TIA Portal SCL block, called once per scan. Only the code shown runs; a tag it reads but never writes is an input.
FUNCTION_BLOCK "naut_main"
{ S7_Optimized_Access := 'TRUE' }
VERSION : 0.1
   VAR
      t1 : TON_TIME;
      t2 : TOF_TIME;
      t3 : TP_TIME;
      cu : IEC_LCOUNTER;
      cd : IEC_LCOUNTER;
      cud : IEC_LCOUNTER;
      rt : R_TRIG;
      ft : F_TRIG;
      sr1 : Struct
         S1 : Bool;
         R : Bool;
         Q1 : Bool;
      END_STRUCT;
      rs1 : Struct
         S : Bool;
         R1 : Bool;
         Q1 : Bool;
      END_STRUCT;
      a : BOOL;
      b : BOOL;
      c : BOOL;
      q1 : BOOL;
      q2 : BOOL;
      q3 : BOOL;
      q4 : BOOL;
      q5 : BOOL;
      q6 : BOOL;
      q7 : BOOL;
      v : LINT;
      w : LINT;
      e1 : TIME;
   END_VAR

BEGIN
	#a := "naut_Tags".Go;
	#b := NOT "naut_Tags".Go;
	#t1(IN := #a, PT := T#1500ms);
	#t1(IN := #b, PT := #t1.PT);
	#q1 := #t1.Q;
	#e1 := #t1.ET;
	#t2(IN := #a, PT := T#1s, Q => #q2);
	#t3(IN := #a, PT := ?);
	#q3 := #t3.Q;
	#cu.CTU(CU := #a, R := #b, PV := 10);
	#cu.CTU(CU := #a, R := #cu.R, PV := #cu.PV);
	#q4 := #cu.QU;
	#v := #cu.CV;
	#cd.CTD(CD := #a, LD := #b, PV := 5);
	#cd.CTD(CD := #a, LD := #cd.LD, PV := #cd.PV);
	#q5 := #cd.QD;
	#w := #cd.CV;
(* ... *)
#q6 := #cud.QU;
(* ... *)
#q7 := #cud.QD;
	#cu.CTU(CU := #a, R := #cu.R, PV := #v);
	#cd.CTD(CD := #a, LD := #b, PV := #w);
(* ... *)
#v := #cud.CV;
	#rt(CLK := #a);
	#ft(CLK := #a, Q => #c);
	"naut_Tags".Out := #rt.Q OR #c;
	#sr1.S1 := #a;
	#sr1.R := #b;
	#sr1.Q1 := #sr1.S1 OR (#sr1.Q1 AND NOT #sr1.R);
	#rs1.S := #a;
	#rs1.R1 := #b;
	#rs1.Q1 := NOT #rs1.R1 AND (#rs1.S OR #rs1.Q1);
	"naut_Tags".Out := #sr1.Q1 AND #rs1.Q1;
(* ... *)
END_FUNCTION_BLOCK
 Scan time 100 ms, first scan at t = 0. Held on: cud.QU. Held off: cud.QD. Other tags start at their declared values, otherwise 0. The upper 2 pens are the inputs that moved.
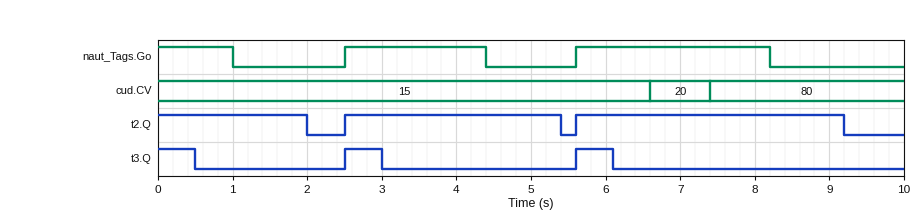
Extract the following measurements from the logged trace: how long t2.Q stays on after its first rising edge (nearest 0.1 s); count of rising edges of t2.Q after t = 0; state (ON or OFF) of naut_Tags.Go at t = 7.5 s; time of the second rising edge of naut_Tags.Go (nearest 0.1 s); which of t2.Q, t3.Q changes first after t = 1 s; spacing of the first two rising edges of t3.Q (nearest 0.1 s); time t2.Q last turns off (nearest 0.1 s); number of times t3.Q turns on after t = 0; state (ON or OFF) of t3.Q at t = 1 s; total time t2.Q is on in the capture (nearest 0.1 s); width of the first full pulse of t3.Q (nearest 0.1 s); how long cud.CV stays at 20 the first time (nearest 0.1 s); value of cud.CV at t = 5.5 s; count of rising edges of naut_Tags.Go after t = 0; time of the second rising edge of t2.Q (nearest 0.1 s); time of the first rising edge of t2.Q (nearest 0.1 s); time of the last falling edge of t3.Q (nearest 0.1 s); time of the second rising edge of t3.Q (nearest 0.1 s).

2.9 s
2
ON
5.6 s
t2.Q
3.1 s
9.2 s
2
OFF
8.5 s
0.5 s
0.8 s
15
2
5.6 s
2.5 s
6.1 s
5.6 s
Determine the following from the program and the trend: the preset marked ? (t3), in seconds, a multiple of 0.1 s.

0.5 s
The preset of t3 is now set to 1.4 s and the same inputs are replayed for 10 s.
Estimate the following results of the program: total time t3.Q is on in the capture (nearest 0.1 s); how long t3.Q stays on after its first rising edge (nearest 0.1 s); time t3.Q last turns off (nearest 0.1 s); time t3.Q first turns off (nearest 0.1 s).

4.2 s
1.4 s
7.0 s
1.4 s
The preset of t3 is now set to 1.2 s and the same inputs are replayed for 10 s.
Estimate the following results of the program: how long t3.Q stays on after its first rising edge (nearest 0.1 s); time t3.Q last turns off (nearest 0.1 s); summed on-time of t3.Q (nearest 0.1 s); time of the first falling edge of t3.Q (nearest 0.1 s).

1.2 s
6.8 s
3.6 s
1.2 s
